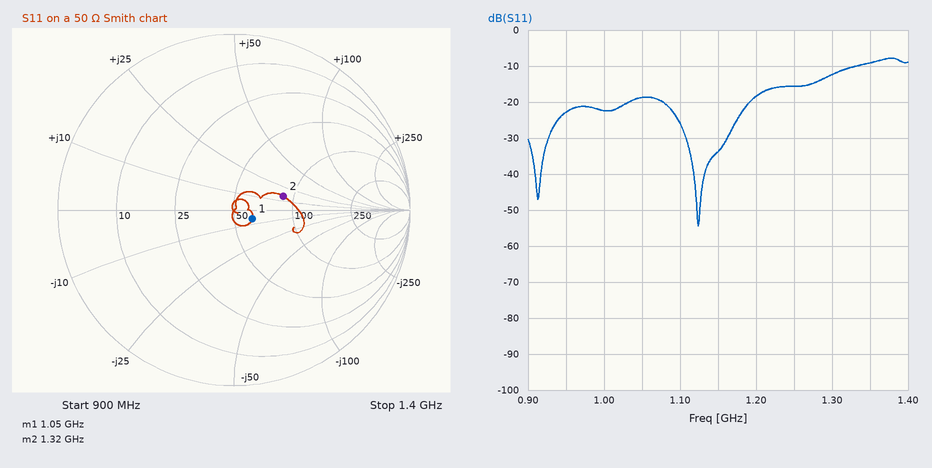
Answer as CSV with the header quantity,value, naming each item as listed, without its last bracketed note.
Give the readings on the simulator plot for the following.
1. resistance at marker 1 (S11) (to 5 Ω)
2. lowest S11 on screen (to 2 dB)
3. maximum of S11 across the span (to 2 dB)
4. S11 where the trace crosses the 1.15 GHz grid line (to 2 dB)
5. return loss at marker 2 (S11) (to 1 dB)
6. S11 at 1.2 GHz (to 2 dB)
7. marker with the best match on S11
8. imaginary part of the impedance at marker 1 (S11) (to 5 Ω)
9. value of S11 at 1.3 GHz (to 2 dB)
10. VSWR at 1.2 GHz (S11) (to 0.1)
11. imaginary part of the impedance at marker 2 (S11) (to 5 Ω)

quantity,value
resistance at marker 1 (S11),60 Ω
lowest S11 on screen,-54 dB
maximum of S11 across the span,-8 dB
S11 where the trace crosses the 1.15 GHz grid line,-34 dB
return loss at marker 2 (S11),11 dB
S11 at 1.2 GHz,-18 dB
marker with the best match on S11,marker 1
imaginary part of the impedance at marker 1 (S11),-5 Ω
value of S11 at 1.3 GHz,-12 dB
VSWR at 1.2 GHz (S11),1.3
imaginary part of the impedance at marker 2 (S11),+15 Ω
